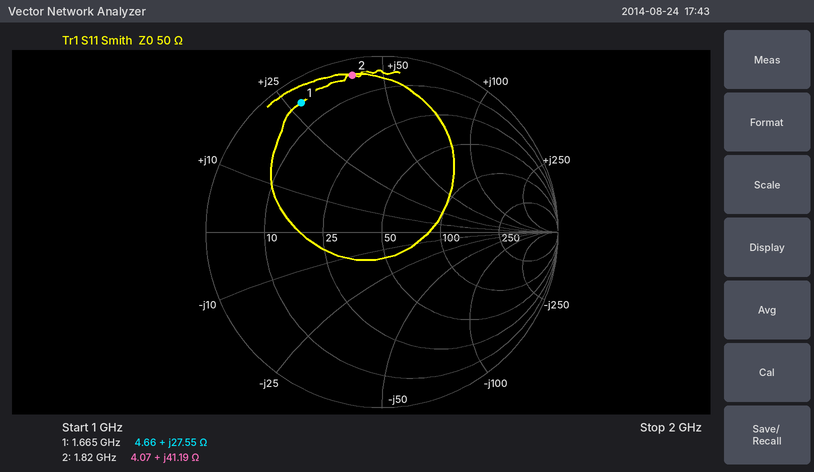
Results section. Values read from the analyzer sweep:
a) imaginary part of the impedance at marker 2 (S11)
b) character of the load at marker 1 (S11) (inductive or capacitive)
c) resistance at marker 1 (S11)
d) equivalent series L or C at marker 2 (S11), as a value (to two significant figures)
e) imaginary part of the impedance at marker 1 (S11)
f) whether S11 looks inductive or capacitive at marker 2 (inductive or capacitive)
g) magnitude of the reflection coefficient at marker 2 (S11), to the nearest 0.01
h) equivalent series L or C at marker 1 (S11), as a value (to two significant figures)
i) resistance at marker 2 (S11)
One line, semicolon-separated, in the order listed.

+41.19 Ω; inductive; 4.66 Ω; 3.6 nH; +27.55 Ω; inductive; 0.91; 2.6 nH; 4.07 Ω
